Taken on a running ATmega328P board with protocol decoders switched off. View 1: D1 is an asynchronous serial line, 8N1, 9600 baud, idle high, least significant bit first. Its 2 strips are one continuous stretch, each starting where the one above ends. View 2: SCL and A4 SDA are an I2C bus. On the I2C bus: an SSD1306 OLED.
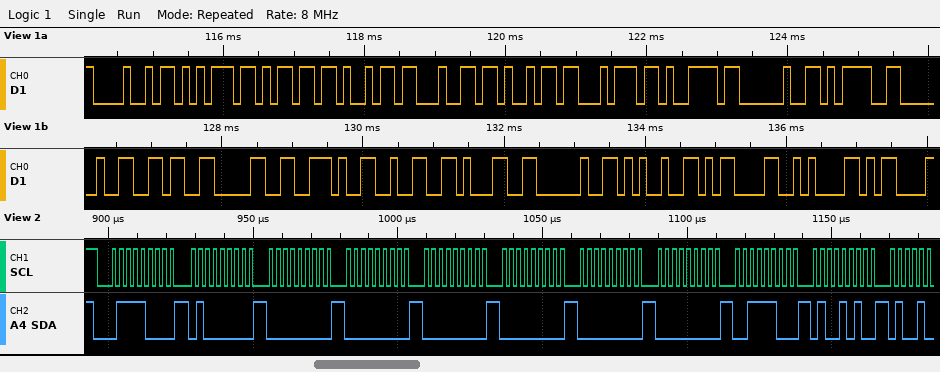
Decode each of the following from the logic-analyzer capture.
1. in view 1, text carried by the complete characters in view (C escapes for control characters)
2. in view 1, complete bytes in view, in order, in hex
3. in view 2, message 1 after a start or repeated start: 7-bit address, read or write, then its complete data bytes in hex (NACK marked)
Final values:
"Humidity = 60.21 %\r\n\r"
48 75 6D 69 64 69 74 79 20 3D 20 36 30 2E 32 31 20 25 0D 0A 0D
0x3C write: 40 00 00 00 00 00 00 3C 4A
